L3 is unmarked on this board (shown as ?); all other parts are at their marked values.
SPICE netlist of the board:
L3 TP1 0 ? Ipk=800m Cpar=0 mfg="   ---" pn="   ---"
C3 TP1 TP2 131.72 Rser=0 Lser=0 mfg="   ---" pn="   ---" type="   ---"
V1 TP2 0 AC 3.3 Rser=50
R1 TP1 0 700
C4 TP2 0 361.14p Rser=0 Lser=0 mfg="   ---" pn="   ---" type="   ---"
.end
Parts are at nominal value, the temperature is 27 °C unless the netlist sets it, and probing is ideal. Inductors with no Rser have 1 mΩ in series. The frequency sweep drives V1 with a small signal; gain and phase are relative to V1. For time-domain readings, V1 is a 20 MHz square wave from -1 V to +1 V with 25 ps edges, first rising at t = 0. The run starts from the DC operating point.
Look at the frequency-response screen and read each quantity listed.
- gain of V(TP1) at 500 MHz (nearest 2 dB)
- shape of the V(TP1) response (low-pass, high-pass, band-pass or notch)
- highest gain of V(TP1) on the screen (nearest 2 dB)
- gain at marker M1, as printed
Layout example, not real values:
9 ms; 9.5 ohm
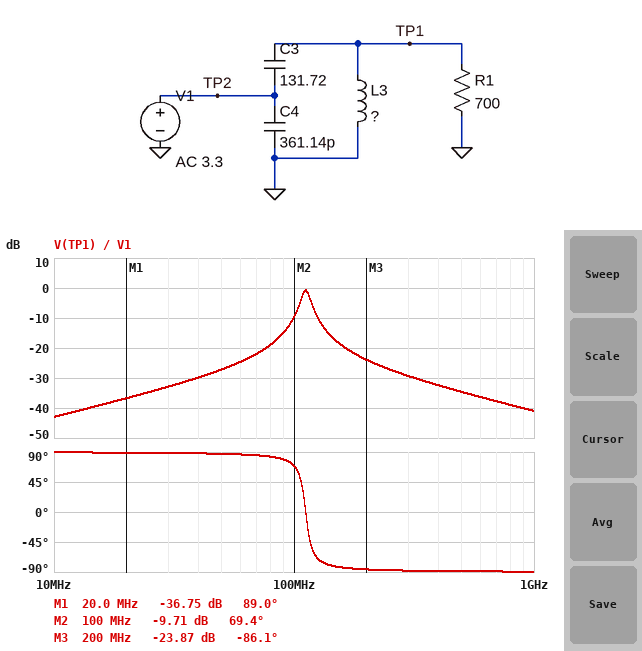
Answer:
-34 dB; band-pass; 0 dB; -36.75 dB
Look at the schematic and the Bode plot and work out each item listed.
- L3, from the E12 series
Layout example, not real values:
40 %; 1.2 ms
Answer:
5.6 nH
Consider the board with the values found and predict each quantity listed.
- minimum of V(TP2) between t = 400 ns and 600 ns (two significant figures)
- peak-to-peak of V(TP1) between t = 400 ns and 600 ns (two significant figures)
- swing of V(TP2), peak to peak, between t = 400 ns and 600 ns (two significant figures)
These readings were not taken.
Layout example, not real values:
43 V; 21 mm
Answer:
-1.1 V; 250 mV; 250 mV
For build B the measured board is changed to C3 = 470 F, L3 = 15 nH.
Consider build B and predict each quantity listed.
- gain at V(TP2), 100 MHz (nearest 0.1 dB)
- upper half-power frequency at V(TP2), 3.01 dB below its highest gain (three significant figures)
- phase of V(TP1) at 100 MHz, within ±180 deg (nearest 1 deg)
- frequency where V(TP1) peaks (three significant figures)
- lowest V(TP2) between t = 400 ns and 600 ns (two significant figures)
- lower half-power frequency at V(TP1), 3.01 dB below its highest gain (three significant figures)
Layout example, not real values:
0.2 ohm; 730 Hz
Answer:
-15.8 dB; 73.3 MHz; -80 deg; 68.4 MHz; -1.2 V; 63.8 MHz
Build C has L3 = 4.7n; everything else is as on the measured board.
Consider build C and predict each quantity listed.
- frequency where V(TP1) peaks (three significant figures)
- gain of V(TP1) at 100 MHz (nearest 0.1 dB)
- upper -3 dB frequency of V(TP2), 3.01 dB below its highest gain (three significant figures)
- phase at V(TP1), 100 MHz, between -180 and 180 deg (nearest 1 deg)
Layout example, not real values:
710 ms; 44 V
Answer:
122 MHz; -15.1 dB; 127 MHz; 79 deg
